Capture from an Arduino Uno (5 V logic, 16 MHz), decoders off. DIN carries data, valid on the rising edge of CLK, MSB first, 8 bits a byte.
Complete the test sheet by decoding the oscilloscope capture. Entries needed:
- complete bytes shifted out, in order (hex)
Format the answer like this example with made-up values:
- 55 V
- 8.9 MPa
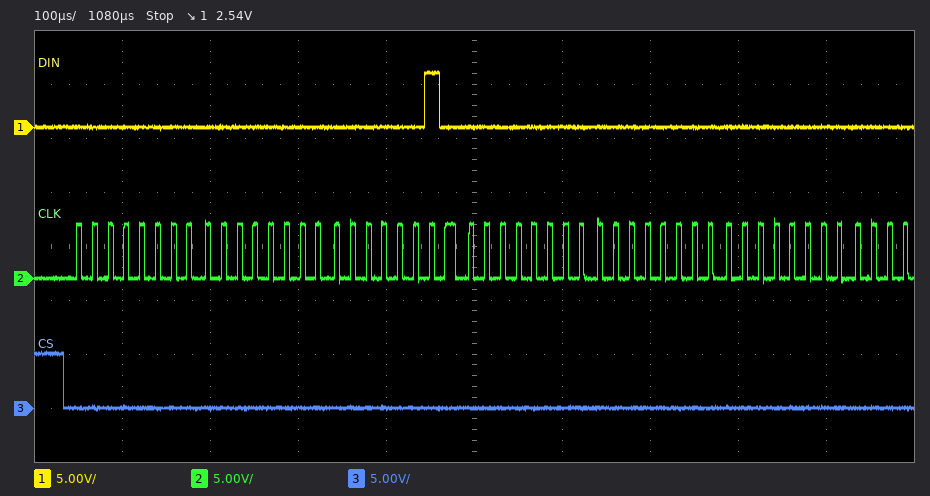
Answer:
- 00 00 02 00 00 00
